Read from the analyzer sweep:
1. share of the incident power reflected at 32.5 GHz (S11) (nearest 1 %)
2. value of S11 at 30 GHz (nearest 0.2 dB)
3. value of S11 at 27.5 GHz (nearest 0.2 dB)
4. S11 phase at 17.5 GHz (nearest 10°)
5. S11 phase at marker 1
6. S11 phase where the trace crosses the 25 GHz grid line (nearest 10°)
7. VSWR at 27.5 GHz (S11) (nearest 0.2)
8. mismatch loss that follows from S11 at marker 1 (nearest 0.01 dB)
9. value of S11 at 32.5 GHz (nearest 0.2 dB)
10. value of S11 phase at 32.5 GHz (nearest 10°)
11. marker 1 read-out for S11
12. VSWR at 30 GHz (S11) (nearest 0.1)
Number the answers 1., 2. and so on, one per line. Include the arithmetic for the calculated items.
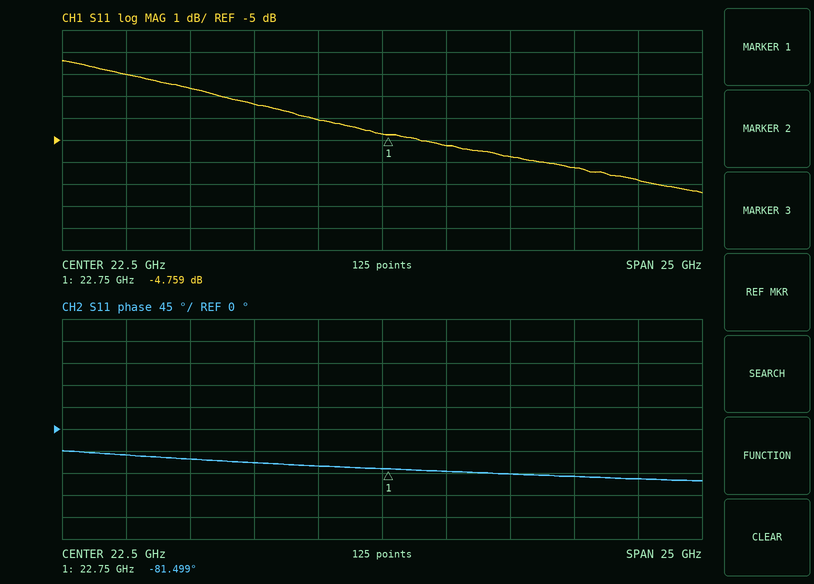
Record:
1. 10^(-6.8/10) ≈ 21 %
2. -6.2 dB
3. -5.8 dB
4. -70°
5. -81.499°
6. -90°
7. |Γ| = 10^(-5.8/20) = 0.5129; VSWR = (1 + 0.5129)/(1 − 0.5129) ≈ 3.11, so 3.2 to the nearest 0.2
8. −10 log10(1 − 10^(-4.759/10)) ≈ 1.77 dB
9. -6.8 dB
10. -100°
11. -4.759 dB
12. |Γ| = 10^(-6.2/20) = 0.4898; VSWR = (1 + 0.4898)/(1 − 0.4898) ≈ 2.9
